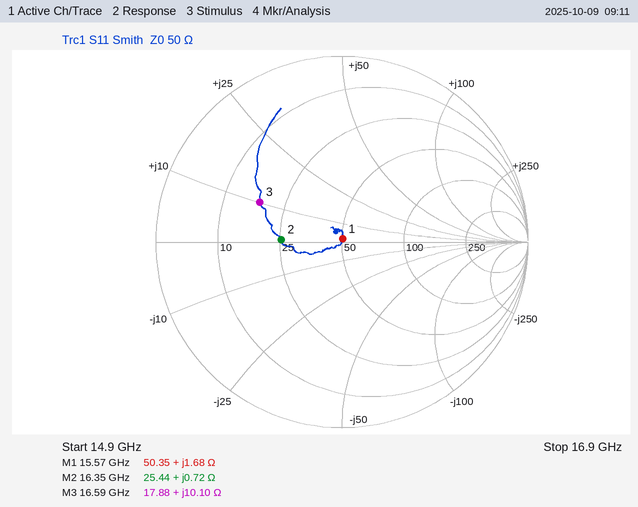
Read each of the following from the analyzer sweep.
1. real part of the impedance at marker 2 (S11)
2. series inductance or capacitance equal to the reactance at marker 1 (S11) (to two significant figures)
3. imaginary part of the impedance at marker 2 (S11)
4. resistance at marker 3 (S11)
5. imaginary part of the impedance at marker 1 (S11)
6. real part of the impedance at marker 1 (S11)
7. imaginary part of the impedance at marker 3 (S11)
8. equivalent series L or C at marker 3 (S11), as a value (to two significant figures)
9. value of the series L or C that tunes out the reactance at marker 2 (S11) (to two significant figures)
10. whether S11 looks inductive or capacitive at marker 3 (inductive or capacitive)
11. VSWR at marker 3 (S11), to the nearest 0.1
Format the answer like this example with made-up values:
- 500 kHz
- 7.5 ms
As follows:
- 25.44 Ω
- 17 pH
- +0.72 Ω
- 17.88 Ω
- +1.68 Ω
- 50.35 Ω
- +10.10 Ω
- 97 pH
- 14 pF
- inductive
- 2.9
